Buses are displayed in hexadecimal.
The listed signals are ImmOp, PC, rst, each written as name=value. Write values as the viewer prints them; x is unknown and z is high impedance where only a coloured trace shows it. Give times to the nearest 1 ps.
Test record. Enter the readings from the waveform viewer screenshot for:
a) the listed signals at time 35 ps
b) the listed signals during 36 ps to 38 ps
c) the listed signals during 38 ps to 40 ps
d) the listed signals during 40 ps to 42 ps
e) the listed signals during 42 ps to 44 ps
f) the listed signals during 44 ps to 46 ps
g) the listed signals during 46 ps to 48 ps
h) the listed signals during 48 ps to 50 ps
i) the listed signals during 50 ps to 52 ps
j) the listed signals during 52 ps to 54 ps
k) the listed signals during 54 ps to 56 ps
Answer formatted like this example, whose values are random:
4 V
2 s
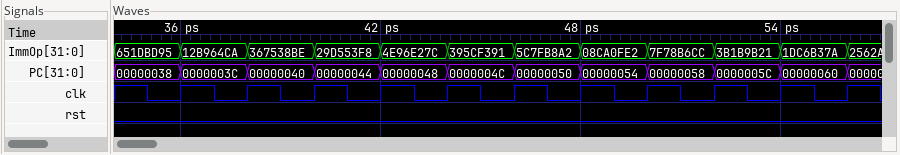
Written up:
ImmOp=651DBD95, PC=00000038, rst=0
ImmOp=12B964CA, PC=0000003C, rst=0
ImmOp=367538BE, PC=00000040, rst=0
ImmOp=29D553F8, PC=00000044, rst=0
ImmOp=4E96E27C, PC=00000048, rst=0
ImmOp=395CF391, PC=0000004C, rst=0
ImmOp=5C7FB8A2, PC=00000050, rst=0
ImmOp=08CA0FE2, PC=00000054, rst=0
ImmOp=7F78B6CC, PC=00000058, rst=0
ImmOp=3B1B9B21, PC=0000005C, rst=0
ImmOp=1DC6B37A, PC=00000060, rst=0
